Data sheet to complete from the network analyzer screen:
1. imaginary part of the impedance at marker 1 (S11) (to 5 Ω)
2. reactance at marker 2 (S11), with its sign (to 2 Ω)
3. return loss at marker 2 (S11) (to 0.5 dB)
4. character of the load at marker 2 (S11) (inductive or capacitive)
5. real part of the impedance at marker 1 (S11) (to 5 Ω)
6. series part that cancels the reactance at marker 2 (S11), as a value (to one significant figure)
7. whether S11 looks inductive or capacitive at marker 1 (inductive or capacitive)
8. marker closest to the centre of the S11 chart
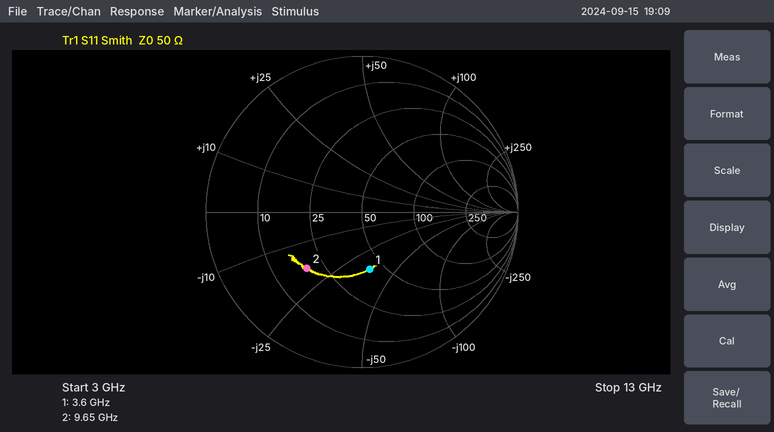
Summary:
-35 Ω
-18 Ω
6.0 dB
capacitive
40 Ω
300 pH
capacitive
marker 1
